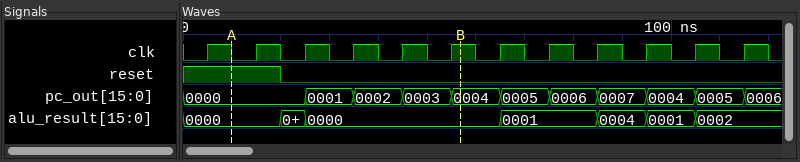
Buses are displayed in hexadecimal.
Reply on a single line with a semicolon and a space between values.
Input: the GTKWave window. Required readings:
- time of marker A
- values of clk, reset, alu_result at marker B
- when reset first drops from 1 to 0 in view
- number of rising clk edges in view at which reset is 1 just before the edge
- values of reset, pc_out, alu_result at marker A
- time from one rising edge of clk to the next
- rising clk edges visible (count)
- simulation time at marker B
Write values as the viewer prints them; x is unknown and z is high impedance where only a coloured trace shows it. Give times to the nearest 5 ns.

10 ns; clk=1, reset=0, alu_result=0000; 20 ns; 2; reset=1, pc_out=0000, alu_result=0000; 10 ns; 12; 55 ns
